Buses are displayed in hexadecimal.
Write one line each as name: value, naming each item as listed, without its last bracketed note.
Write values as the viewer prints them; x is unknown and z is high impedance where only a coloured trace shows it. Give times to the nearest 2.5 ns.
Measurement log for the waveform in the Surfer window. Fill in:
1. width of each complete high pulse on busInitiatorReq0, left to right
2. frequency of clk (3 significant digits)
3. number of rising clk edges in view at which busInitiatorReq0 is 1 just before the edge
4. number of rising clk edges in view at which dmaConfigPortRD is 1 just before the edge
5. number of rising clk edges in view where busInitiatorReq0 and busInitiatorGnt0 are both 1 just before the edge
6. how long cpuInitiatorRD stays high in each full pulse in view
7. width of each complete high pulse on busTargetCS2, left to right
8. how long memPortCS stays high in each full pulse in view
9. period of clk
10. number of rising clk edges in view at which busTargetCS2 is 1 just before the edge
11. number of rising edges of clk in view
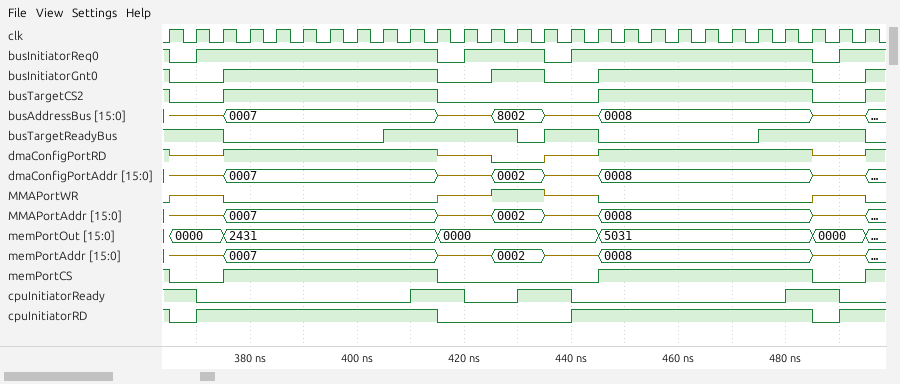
width of each complete high pulse on busInitiatorReq0, left to right: 45 ns, 15 ns, 45 ns
frequency of clk: 200 MHz
number of rising clk edges in view at which busInitiatorReq0 is 1 just before the edge: 23
number of rising clk edges in view at which dmaConfigPortRD is 1 just before the edge: 17
number of rising clk edges in view where busInitiatorReq0 and busInitiatorGnt0 are both 1 just before the edge: 19
how long cpuInitiatorRD stays high in each full pulse in view: 45 ns, 45 ns
width of each complete high pulse on busTargetCS2, left to right: 40 ns, 40 ns
how long memPortCS stays high in each full pulse in view: 40 ns, 40 ns
period of clk: 5 ns
number of rising clk edges in view at which busTargetCS2 is 1 just before the edge: 17
number of rising edges of clk in view: 27
